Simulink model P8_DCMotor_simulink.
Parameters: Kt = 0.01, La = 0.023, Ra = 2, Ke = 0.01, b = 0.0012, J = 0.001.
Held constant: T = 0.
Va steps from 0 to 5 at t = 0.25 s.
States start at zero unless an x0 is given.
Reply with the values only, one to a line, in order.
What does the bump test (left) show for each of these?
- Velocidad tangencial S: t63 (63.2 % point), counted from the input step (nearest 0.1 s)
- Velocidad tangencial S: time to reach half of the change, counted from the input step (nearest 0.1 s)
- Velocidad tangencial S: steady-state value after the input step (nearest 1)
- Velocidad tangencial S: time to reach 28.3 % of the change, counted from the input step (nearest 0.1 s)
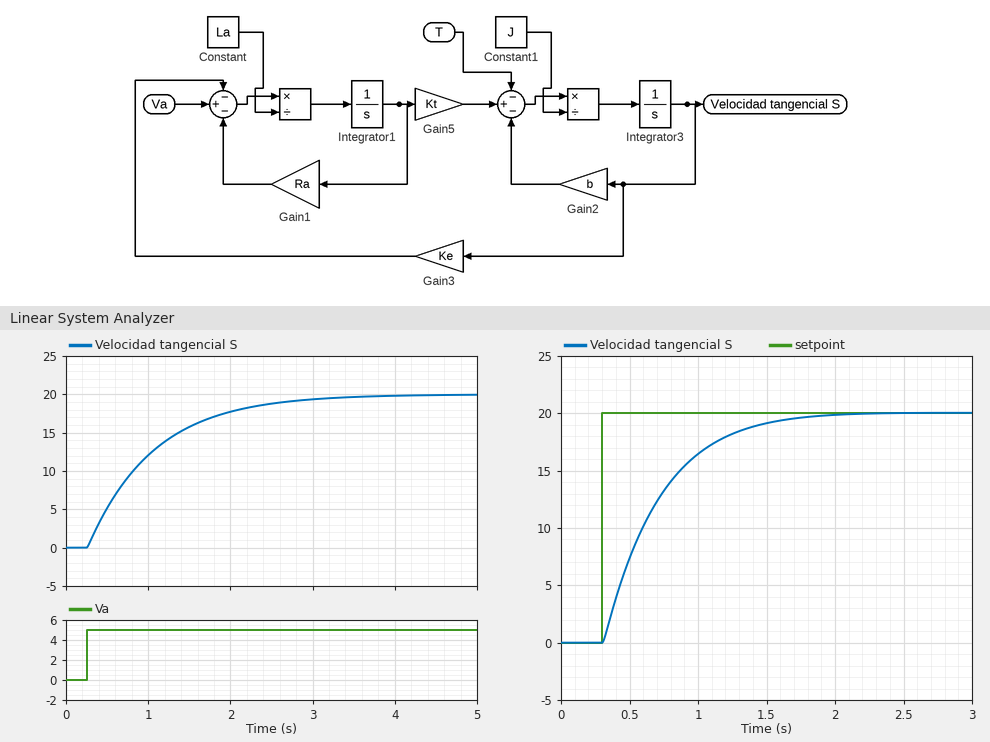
0.8 s
0.6 s
20
0.3 s
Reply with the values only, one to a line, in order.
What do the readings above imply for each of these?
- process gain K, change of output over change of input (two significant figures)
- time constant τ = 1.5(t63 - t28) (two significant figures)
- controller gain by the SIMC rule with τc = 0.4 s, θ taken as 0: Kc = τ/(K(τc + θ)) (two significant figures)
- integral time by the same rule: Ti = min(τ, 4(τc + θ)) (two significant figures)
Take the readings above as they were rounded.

4.0
0.75 s
0.47
0.75 s
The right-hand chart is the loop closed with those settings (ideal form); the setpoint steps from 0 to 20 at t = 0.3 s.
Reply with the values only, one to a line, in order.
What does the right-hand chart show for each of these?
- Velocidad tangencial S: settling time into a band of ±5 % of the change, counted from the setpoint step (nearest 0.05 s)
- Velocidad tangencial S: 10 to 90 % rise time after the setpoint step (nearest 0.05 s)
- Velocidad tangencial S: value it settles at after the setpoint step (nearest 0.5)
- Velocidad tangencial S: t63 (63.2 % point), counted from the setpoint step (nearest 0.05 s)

1.15 s
0.85 s
20.0
0.40 s
